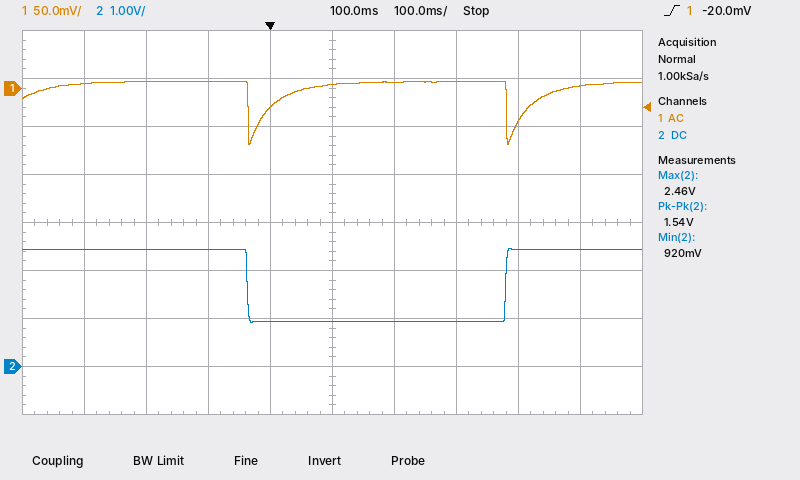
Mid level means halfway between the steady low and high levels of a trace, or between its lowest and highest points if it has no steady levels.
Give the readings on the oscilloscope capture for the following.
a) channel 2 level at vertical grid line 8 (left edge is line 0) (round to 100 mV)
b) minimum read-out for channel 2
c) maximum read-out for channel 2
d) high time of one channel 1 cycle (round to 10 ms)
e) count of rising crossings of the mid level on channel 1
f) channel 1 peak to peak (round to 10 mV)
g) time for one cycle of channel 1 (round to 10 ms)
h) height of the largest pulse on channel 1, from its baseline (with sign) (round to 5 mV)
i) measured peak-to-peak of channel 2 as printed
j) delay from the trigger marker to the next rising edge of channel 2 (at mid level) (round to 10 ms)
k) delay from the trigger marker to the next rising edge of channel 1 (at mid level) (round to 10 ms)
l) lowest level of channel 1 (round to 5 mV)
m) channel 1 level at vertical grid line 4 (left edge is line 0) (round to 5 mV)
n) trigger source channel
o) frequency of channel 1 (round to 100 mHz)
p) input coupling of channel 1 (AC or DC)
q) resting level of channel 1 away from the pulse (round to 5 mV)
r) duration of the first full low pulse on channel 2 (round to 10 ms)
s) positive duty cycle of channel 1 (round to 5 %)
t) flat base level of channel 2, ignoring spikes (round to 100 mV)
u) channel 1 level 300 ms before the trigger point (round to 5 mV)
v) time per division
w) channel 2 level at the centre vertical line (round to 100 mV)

2.4 V
920 mV
2.46 V
390 ms
2
70 mV
420 ms
-65 mV
1.54 V
380 ms
410 ms
-60 mV
-20 mV
channel 1
2.4 Hz
AC
5 mV
420 ms
95 %
900 mV
5 mV
100 ms
900 mV
